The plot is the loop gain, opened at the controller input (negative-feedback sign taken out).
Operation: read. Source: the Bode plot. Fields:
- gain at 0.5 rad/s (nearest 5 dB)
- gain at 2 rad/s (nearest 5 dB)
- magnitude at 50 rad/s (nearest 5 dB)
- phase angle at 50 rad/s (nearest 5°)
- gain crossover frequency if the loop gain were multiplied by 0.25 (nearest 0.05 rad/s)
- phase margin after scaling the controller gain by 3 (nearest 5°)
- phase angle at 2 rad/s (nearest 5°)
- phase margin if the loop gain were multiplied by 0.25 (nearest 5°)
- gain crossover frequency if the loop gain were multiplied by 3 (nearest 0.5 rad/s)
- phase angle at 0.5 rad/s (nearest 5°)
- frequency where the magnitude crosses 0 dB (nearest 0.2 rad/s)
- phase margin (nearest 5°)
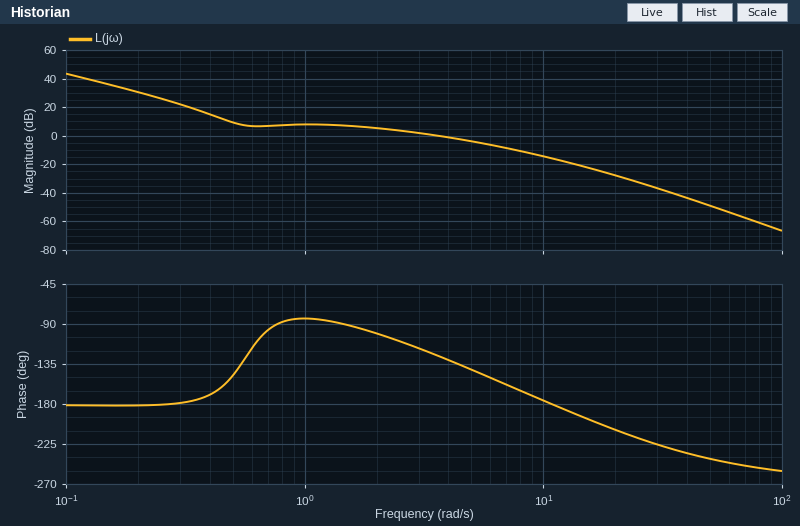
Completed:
10 dB
5 dB
-50 dB
-240°
0.45 rad/s
20°
-100°
20°
7.5 rad/s
-150°
3.6 rad/s
55°
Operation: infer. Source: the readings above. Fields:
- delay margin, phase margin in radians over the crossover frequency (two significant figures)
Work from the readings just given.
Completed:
0.27 s
